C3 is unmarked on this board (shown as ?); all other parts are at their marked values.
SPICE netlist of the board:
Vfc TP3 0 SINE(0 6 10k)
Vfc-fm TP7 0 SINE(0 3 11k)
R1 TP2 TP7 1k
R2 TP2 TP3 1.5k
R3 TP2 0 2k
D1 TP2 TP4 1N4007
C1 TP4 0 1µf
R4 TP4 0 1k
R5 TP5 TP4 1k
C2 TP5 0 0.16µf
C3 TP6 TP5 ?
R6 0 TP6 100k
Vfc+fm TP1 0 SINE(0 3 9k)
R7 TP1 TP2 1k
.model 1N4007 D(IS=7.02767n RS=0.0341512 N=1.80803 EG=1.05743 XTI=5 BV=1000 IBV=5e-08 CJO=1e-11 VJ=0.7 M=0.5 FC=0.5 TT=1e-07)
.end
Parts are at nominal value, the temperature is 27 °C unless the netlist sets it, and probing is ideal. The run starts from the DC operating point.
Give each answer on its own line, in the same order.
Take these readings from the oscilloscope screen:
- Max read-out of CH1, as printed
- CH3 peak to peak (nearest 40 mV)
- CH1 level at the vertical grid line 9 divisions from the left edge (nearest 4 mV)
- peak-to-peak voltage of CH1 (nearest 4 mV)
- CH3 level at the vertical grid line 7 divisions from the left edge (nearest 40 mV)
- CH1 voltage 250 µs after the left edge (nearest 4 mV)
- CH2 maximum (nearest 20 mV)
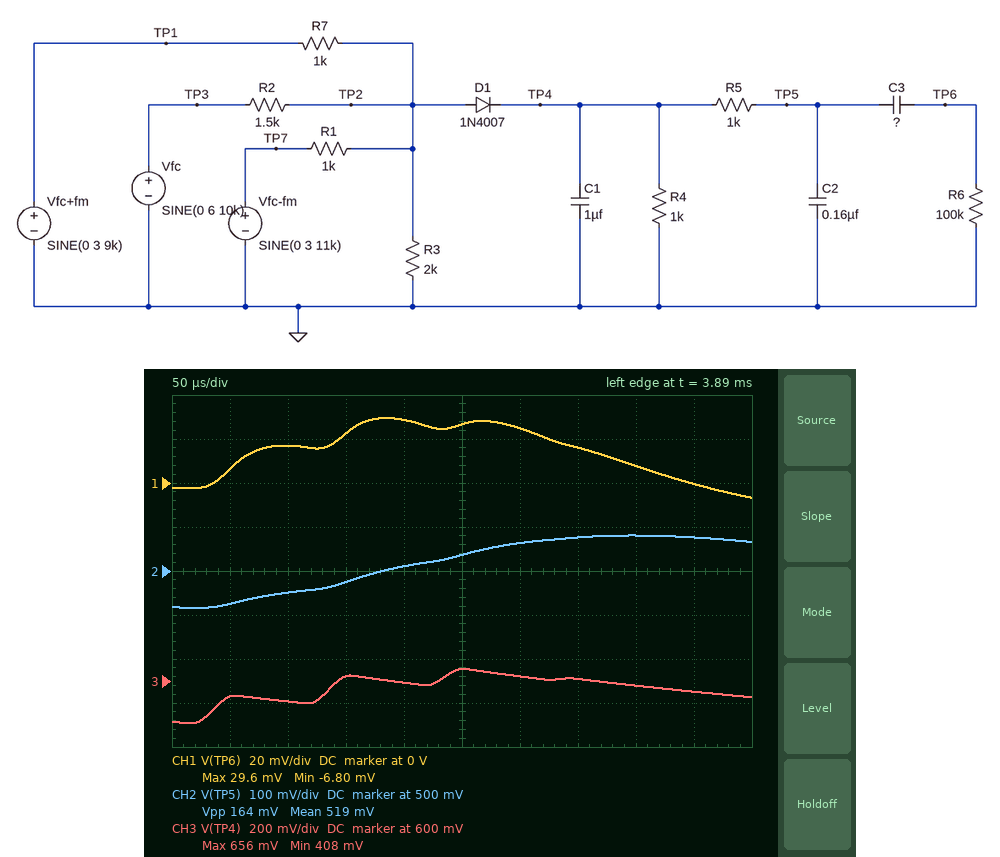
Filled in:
29.6 mV
240 mV
0 V
36 mV
600 mV
28 mV
580 mV
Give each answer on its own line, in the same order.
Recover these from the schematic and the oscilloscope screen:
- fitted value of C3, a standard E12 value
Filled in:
470 pF
